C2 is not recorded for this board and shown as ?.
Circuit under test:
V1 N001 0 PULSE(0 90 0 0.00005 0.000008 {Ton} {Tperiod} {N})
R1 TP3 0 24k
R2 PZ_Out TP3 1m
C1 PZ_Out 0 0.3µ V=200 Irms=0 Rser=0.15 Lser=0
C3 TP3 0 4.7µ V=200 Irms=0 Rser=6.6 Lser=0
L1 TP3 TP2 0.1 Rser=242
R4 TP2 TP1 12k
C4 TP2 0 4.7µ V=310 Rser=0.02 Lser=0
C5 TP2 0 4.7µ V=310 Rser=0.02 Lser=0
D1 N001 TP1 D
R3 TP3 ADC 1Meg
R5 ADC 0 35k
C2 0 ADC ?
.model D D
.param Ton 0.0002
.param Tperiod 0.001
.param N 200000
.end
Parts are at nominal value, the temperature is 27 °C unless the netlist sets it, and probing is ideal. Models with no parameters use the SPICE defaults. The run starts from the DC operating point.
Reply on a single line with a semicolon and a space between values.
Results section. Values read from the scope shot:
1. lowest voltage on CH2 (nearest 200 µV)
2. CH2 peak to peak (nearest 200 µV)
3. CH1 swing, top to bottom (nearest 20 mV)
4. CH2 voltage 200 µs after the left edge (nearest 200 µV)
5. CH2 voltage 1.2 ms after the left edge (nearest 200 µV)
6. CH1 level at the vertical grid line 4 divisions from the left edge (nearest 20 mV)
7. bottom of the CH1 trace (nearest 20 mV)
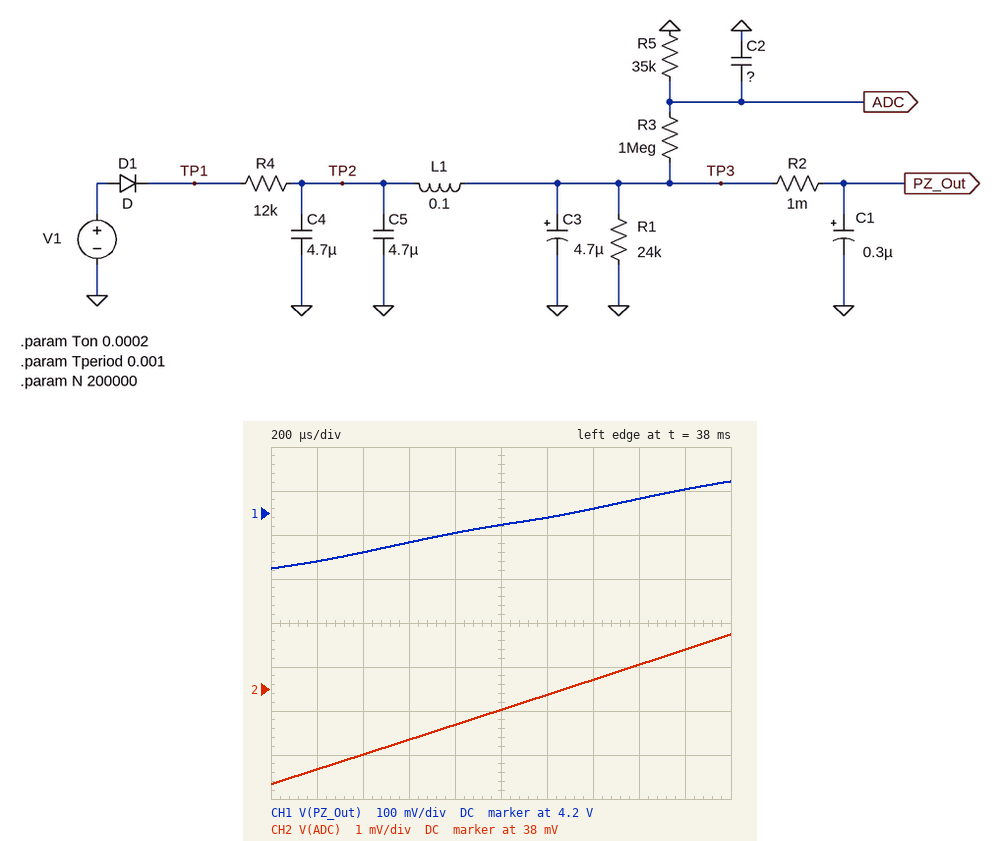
35.8 mV; 3.4 mV; 200 mV; 36.2 mV; 37.8 mV; 4.16 V; 4.08 V
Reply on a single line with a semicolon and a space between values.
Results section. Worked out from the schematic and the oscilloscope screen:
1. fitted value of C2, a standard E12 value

1.8 µF
